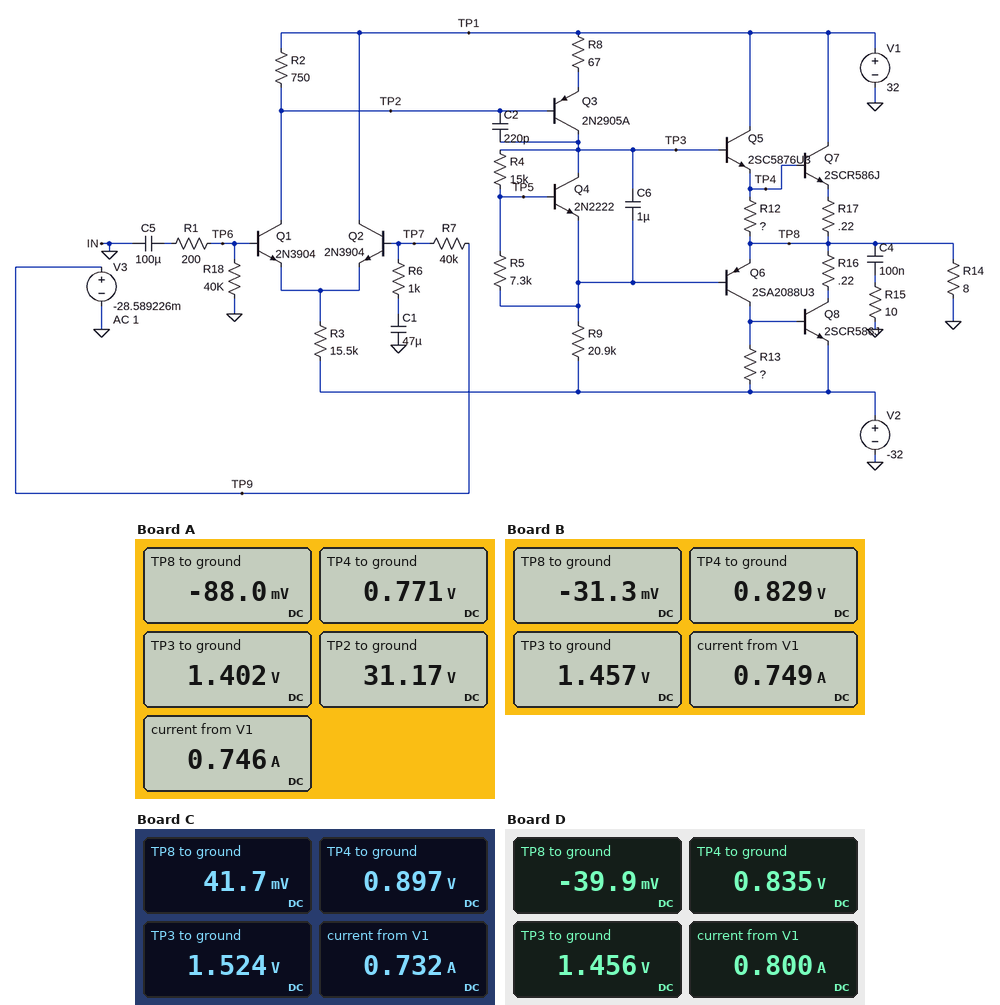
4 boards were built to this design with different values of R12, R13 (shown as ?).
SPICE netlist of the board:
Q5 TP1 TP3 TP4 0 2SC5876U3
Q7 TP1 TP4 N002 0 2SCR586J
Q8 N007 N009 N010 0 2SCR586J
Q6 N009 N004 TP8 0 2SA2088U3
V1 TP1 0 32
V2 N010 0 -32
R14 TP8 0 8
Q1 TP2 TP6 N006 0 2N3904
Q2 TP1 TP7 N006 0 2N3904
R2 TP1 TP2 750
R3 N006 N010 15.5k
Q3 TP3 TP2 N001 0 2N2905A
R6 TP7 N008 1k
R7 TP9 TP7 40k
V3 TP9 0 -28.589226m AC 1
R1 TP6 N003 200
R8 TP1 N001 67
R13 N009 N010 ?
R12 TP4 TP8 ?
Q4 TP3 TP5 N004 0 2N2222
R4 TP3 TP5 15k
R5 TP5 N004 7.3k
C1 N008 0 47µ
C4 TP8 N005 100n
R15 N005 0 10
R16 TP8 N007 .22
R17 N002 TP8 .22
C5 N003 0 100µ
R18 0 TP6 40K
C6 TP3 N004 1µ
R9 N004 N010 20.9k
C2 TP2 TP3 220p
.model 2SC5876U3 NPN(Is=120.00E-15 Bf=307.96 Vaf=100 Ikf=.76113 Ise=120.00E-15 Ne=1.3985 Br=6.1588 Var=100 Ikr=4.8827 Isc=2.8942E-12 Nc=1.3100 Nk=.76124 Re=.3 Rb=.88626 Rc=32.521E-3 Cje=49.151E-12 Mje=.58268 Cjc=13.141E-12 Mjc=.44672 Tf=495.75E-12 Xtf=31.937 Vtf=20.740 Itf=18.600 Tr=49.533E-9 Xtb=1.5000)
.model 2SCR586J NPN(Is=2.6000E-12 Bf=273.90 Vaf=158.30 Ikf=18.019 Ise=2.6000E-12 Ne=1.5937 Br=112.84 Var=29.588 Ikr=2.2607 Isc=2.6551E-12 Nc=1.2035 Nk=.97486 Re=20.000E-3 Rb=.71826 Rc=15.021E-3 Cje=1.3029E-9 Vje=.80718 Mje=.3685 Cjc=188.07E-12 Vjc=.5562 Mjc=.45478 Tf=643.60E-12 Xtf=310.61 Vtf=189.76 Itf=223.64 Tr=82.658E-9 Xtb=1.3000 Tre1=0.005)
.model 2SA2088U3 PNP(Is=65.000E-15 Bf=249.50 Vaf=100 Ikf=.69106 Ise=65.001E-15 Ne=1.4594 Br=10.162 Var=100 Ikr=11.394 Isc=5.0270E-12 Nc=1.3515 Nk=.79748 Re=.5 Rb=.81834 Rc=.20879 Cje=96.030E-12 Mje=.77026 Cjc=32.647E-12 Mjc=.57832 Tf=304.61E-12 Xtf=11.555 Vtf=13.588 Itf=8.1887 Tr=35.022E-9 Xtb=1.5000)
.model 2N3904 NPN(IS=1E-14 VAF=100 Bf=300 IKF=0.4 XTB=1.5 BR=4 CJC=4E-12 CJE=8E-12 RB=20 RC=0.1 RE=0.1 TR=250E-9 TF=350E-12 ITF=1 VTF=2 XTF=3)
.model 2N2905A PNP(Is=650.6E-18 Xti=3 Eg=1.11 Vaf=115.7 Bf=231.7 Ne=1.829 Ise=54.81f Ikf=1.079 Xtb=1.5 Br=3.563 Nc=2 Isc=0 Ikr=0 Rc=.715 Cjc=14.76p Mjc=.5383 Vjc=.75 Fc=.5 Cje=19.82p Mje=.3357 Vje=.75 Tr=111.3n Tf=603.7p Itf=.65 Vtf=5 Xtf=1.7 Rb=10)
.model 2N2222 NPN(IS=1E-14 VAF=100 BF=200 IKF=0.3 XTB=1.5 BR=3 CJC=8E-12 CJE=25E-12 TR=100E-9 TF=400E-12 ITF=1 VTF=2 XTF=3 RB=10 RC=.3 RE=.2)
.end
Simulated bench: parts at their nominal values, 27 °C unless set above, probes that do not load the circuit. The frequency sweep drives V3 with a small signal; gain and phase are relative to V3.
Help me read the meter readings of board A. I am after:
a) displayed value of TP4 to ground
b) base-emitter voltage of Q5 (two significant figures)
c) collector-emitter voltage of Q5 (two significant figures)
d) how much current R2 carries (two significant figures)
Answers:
0.771 V
630 mV
31 V
1.1 mA
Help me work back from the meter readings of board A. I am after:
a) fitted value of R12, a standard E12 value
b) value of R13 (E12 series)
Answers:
270 Ω
390 Ω
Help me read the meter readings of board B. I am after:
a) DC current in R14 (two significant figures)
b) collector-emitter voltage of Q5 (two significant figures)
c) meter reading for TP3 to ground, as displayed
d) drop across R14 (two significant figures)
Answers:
3.9 mA
31 V
1.457 V
31 mV
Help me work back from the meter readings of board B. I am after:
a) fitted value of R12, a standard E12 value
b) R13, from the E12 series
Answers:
330 Ω
330 Ω
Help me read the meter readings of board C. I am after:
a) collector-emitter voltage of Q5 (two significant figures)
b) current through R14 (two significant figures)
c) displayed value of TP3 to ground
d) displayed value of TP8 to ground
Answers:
31 V
5.2 mA
1.524 V
41.7 mV
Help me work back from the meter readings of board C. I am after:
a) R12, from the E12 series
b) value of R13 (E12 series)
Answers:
330 Ω
220 Ω
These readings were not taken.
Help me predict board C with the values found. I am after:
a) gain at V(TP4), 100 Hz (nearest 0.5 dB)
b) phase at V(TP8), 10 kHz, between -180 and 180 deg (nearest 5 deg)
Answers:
37.0 dB
110 deg
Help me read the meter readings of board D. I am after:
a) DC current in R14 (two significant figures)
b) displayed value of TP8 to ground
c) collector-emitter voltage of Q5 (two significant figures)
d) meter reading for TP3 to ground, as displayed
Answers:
5.0 mA
-39.9 mV
31 V
1.456 V
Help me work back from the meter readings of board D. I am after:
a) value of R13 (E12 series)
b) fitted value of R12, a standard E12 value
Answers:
820 Ω
680 Ω
